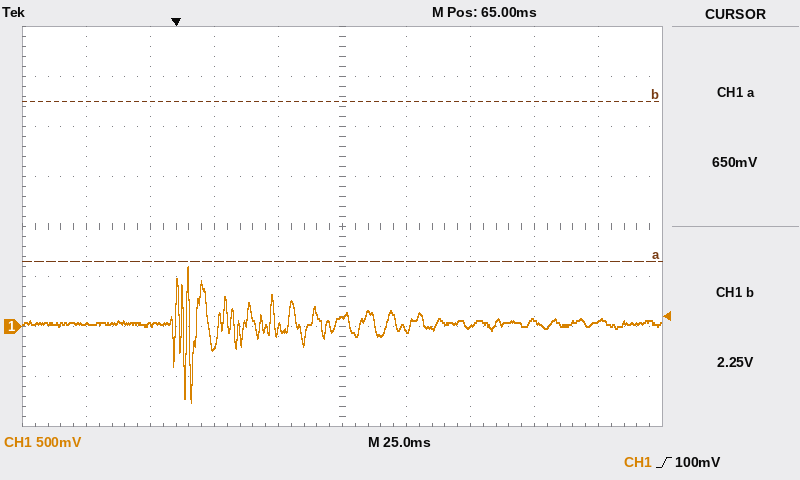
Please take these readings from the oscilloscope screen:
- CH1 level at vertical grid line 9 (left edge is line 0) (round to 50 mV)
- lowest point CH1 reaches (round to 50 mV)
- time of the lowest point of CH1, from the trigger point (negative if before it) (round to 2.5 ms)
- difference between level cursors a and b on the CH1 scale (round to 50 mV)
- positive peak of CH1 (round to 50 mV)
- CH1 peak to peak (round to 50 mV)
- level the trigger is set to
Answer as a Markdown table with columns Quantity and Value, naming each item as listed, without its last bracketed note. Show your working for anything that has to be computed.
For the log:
| Quantity | Value |
|---|---|
| CH1 level at vertical grid line 9 (left edge is line 0) | 50 mV |
| lowest point CH1 reaches | -750 mV |
| time of the lowest point of CH1, from the trigger point (negative if before it) | +5.0 ms |
| difference between level cursors a and b on the CH1 scale | 1.60 V |
| positive peak of CH1 | 600 mV |
| CH1 peak to peak | 600 mV − (-750 mV) = 1.35 V |
| level the trigger is set to | 100 mV |
